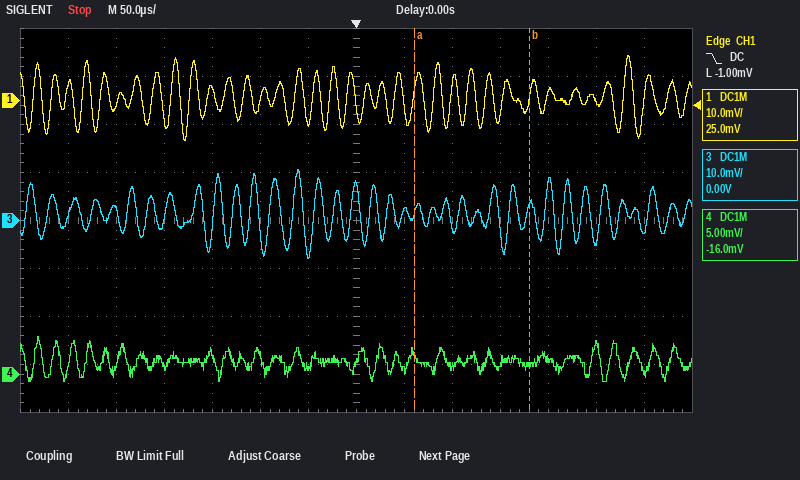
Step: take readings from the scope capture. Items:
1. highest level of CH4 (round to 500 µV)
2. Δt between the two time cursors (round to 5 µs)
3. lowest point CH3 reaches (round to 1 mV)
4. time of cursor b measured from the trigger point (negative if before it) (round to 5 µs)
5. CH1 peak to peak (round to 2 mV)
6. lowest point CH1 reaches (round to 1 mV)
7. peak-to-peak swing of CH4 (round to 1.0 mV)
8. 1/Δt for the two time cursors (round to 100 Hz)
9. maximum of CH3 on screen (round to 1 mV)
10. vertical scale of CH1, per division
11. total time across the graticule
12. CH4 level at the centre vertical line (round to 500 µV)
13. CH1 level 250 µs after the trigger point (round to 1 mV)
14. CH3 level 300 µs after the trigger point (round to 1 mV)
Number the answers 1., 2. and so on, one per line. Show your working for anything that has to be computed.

1. 4.0 mV
2. 120 µs
3. -8 mV
4. +180 µs
5. 18 mV
6. -8 mV
7. 5.0 mV
8. 1 / 120 µs ≈ 8.3 kHz
9. 11 mV
10. 10 mV
11. 700 µs
12. 1.0 mV
13. 0 mV
14. -2 mV
